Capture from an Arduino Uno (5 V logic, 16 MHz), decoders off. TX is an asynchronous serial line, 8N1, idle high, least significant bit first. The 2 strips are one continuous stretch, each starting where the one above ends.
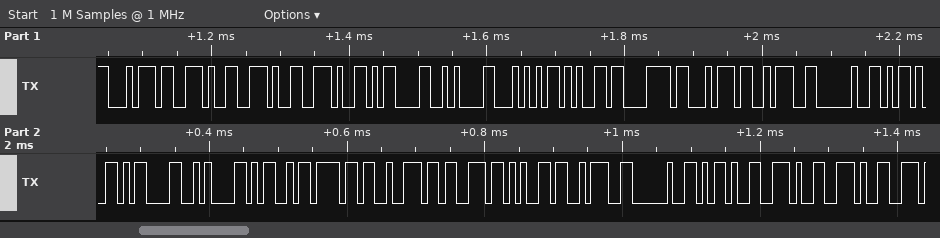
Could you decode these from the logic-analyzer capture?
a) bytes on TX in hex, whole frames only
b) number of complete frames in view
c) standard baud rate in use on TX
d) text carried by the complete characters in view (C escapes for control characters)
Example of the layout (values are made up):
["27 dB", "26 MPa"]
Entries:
["74 2E 2E 2E 0D 0A 54 65 78 74 3A 20 2D 0D 0A 4D 6F 72 73 65 3A 20 2D 2E 2E", "25", "115200 baud", "\"t...\\r\\nText: -\\r\\nMorse: -..\""]
